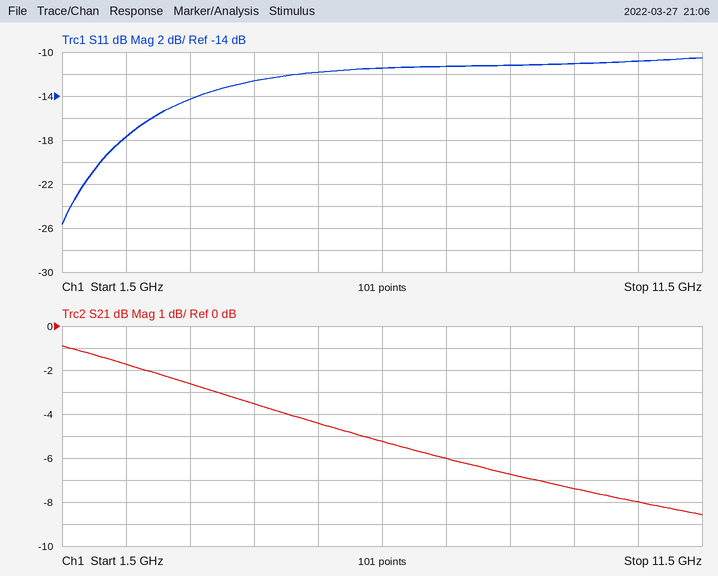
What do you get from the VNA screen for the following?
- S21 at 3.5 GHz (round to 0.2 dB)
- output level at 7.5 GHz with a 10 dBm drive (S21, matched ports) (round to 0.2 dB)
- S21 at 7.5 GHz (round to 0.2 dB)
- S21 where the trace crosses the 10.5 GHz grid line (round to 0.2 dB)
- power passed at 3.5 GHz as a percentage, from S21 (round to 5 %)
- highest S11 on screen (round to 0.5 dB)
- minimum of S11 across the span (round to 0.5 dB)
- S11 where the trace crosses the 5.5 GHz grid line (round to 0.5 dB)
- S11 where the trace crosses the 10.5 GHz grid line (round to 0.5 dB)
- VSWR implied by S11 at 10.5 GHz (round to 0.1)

-2.6 dB
4.0 dBm
-6.0 dB
-8.0 dB
55 %
-10.5 dB
-25.5 dB
-12.0 dB
-11.0 dB
1.8
